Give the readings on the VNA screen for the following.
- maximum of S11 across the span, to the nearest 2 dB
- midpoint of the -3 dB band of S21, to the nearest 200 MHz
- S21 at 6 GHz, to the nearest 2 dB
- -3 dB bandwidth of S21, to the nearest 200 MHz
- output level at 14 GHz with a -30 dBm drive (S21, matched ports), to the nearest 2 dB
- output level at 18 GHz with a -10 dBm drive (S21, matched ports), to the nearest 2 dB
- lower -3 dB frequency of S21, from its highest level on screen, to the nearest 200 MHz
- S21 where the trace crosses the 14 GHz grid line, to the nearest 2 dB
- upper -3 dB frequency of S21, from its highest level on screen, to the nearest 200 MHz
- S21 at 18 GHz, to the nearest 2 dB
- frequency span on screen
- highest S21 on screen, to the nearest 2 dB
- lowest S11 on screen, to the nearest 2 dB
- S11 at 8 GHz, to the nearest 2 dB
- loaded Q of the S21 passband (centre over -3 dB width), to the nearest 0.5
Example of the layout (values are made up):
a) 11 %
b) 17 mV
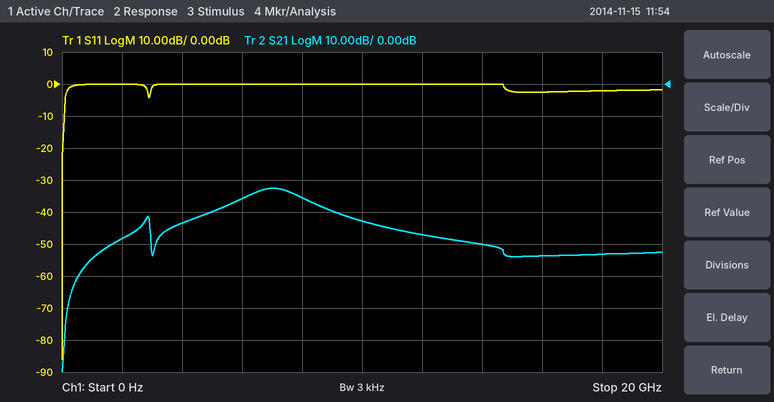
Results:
a) 0 dB
b) 7.0 GHz
c) -36 dB
d) 2.0 GHz
e) -80 dBm
f) -64 dBm
g) 6.0 GHz
h) -50 dB
i) 8.0 GHz
j) -54 dB
k) 20 GHz
l) -32 dB
m) -86 dB
n) 0 dB
o) 3.5
